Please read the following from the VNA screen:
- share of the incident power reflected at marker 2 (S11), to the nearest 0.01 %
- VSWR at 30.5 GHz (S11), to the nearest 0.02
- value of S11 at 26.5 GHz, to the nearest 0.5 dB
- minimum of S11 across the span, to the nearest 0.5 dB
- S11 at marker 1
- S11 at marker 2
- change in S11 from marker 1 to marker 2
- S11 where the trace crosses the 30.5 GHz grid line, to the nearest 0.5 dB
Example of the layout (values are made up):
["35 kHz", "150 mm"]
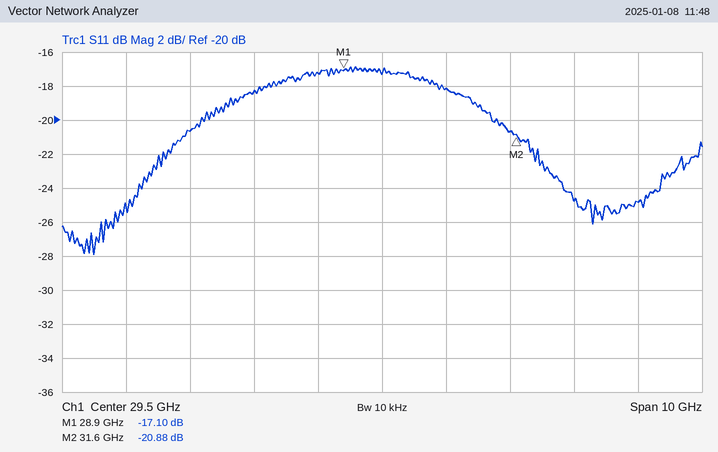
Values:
["0.82 %", "1.28", "-20.5 dB", "-28.0 dB", "-17.10 dB", "-20.88 dB", "-3.78 dB", "-18.0 dB"]
